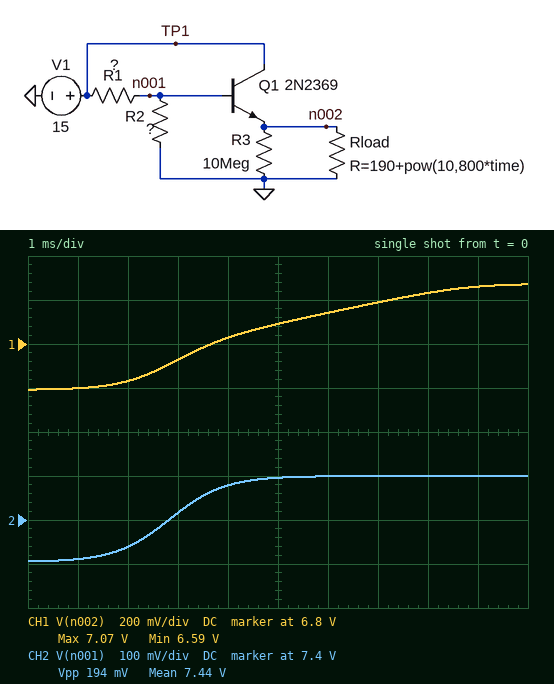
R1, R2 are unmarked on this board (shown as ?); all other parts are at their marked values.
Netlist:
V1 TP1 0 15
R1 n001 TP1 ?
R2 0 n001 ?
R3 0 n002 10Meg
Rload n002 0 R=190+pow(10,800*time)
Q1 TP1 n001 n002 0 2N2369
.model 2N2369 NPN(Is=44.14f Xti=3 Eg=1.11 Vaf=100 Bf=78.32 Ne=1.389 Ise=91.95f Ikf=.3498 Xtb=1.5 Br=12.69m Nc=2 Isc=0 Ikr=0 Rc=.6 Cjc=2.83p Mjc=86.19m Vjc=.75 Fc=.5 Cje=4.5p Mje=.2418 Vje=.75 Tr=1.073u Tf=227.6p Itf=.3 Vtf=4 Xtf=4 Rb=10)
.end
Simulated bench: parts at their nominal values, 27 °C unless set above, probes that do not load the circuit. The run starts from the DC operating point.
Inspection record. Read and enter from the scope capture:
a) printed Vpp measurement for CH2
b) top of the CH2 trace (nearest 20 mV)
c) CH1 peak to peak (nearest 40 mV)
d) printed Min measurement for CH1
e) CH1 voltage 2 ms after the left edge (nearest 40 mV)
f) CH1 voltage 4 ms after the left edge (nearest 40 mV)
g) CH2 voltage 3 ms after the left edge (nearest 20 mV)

194 mV
7.50 V
480 mV
6.59 V
6.64 V
6.84 V
7.42 V
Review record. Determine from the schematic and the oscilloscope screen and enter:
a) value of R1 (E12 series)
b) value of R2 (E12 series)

820 Ω
820 Ω
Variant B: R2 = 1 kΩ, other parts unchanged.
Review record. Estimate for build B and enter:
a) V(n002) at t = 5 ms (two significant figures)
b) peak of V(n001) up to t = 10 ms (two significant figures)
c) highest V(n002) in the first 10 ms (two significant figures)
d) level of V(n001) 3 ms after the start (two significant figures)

7.6 V
8.2 V
7.8 V
8.1 V
